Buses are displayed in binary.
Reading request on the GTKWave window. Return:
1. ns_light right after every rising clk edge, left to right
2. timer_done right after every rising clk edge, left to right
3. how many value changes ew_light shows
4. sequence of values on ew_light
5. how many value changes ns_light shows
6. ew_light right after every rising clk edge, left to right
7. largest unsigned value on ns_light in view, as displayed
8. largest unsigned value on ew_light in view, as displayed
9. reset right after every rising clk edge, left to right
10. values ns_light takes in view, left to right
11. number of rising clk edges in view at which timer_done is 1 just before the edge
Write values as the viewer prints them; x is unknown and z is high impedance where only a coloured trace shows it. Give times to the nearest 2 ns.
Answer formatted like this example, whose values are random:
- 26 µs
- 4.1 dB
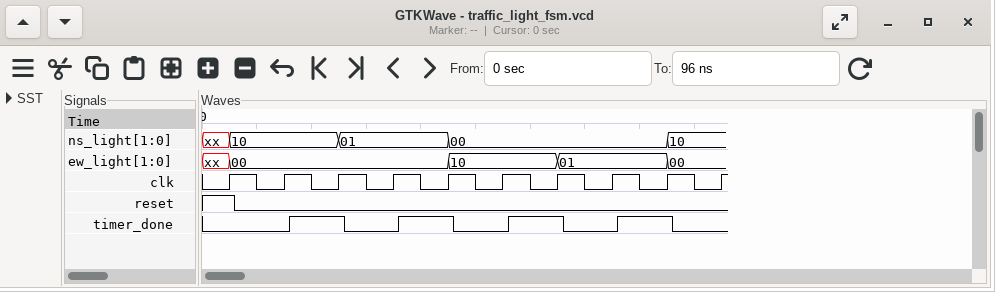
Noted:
- 10, 10, 01, 01, 00, 00, 00, 00, 10, 10
- 0 0 1 0 1 0 1 0 1 0
- 4
- xx, 00, 10, 01, 00
- 4
- 00, 00, 00, 00, 10, 10, 01, 01, 00, 00
- 10
- 10
- 1 0 0 0 0 0 0 0 0 0
- xx, 10, 01, 00, 10
- 4
